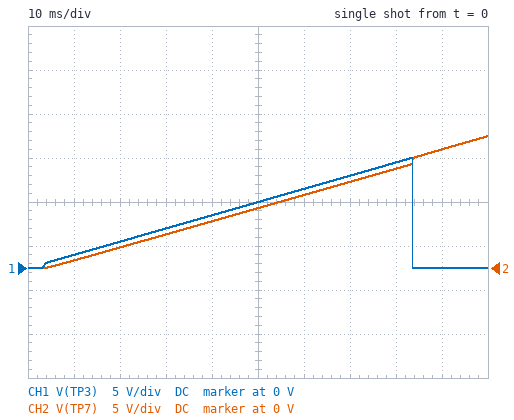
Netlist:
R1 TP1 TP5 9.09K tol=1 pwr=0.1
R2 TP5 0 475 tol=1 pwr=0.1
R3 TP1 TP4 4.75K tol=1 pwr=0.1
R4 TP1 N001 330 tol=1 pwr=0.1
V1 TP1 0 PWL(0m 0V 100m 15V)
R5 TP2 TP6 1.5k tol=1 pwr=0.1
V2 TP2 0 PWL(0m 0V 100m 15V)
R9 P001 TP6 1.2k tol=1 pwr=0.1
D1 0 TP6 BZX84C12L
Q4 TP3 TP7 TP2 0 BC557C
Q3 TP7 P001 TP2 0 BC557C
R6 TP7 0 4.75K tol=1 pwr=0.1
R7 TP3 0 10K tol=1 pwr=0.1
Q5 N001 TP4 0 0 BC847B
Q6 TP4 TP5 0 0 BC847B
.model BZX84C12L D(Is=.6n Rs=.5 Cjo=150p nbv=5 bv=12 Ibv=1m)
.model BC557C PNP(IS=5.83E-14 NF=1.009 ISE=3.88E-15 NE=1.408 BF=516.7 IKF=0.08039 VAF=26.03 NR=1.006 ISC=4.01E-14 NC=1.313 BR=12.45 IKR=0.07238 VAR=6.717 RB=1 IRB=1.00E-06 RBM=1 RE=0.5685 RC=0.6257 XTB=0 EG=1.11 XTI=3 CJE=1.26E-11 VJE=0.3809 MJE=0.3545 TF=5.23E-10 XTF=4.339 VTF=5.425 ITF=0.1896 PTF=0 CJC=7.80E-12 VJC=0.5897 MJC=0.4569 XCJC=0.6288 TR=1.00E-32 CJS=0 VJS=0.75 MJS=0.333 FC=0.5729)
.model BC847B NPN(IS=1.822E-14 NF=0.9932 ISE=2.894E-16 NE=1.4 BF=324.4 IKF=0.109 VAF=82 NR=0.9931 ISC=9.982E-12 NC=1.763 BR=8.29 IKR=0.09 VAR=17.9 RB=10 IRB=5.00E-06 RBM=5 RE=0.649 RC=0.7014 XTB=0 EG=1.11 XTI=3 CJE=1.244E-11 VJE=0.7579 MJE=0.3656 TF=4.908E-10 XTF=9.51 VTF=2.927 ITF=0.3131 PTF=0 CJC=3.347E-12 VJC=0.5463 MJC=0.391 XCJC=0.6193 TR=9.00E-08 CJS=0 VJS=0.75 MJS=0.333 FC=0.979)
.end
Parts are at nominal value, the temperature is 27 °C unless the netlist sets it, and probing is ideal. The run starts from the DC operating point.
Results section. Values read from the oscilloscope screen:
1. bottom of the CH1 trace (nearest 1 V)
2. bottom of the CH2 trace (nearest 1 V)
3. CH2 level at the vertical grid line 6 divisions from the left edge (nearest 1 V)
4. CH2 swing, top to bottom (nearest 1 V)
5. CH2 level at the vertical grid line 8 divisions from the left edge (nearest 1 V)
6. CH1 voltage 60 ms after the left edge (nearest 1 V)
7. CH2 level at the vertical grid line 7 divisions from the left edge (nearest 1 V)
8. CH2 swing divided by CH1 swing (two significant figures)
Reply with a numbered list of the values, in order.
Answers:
1. 0 V
2. 0 V
3. 8 V
4. 15 V
5. 11 V
6. 9 V
7. 10 V
8. 1.2
